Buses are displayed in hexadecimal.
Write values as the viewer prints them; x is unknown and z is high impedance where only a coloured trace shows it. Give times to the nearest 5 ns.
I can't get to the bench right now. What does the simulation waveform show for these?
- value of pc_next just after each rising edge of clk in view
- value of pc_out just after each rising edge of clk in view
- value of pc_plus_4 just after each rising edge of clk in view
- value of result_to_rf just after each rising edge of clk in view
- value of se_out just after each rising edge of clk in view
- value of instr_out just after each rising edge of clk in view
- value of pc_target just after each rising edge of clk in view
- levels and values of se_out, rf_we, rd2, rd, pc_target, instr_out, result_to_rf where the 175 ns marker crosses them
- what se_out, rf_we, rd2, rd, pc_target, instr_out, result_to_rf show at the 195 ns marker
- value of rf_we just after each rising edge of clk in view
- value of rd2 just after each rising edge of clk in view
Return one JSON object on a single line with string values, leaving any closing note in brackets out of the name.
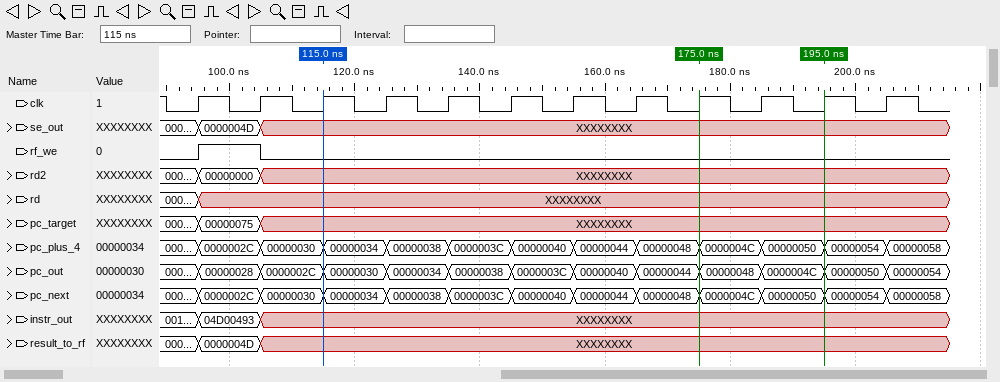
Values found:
{"value of pc_next just after each rising edge of clk in view": "0000002C, 00000030, 00000034, 00000038, 0000003C, 00000040, 00000044, 00000048, 0000004C, 00000050, 00000054, 00000058", "value of pc_out just after each rising edge of clk in view": "00000028, 0000002C, 00000030, 00000034, 00000038, 0000003C, 00000040, 00000044, 00000048, 0000004C, 00000050, 00000054", "value of pc_plus_4 just after each rising edge of clk in view": "0000002C, 00000030, 00000034, 00000038, 0000003C, 00000040, 00000044, 00000048, 0000004C, 00000050, 00000054, 00000058", "value of result_to_rf just after each rising edge of clk in view": "0000004D, XXXXXXXX, XXXXXXXX, XXXXXXXX, XXXXXXXX, XXXXXXXX, XXXXXXXX, XXXXXXXX, XXXXXXXX, XXXXXXXX, XXXXXXXX, XXXXXXXX", "value of se_out just after each rising edge of clk in view": "0000004D, XXXXXXXX, XXXXXXXX, XXXXXXXX, XXXXXXXX, XXXXXXXX, XXXXXXXX, XXXXXXXX, XXXXXXXX, XXXXXXXX, XXXXXXXX, XXXXXXXX", "value of instr_out just after each rising edge of clk in view": "04D00493, XXXXXXXX, XXXXXXXX, XXXXXXXX, XXXXXXXX, XXXXXXXX, XXXXXXXX, XXXXXXXX, XXXXXXXX, XXXXXXXX, XXXXXXXX, XXXXXXXX", "value of pc_target just after each rising edge of clk in view": "00000075, XXXXXXXX, XXXXXXXX, XXXXXXXX, XXXXXXXX, XXXXXXXX, XXXXXXXX, XXXXXXXX, XXXXXXXX, XXXXXXXX, XXXXXXXX, XXXXXXXX", "levels and values of se_out, rf_we, rd2, rd, pc_target, instr_out, result_to_rf where the 175 ns marker crosses them": "se_out=XXXXXXXX, rf_we=0, rd2=XXXXXXXX, rd=XXXXXXXX, pc_target=XXXXXXXX, instr_out=XXXXXXXX, result_to_rf=XXXXXXXX", "what se_out, rf_we, rd2, rd, pc_target, instr_out, result_to_rf show at the 195 ns marker": "se_out=XXXXXXXX, rf_we=0, rd2=XXXXXXXX, rd=XXXXXXXX, pc_target=XXXXXXXX, instr_out=XXXXXXXX, result_to_rf=XXXXXXXX", "value of rf_we just after each rising edge of clk in view": "1 0 0 0 0 0 0 0 0 0 0 0", "value of rd2 just after each rising edge of clk in view": "00000000, XXXXXXXX, XXXXXXXX, XXXXXXXX, XXXXXXXX, XXXXXXXX, XXXXXXXX, XXXXXXXX, XXXXXXXX, XXXXXXXX, XXXXXXXX, XXXXXXXX"}
